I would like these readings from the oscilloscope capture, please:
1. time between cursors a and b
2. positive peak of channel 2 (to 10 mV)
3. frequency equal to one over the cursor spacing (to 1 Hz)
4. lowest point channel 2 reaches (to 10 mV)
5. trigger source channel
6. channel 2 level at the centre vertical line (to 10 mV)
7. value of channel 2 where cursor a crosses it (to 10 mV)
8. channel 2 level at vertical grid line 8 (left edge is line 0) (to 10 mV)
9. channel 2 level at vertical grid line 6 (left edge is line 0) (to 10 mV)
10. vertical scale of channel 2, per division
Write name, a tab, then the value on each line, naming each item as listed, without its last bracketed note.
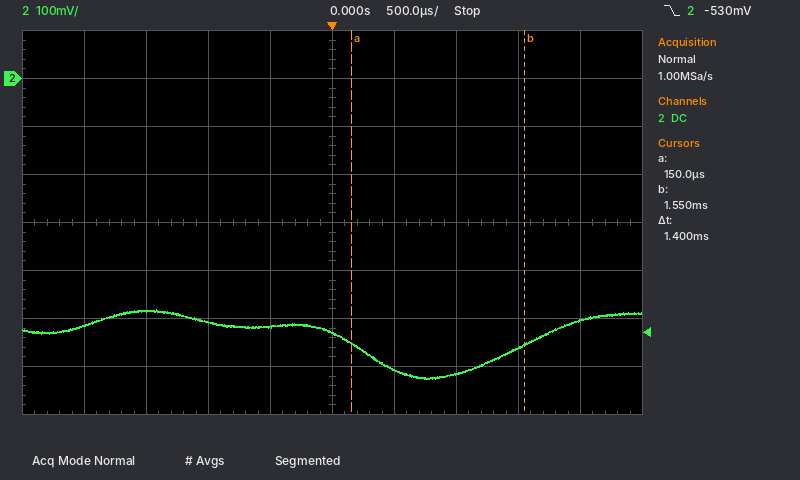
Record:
time between cursors a and b	1.4 ms
positive peak of channel 2	-480 mV
frequency equal to one over the cursor spacing	714 Hz
lowest point channel 2 reaches	-630 mV
trigger source channel	channel 2
channel 2 level at the centre vertical line	-530 mV
value of channel 2 where cursor a crosses it	-550 mV
channel 2 level at vertical grid line 8 (left edge is line 0)	-560 mV
channel 2 level at vertical grid line 6 (left edge is line 0)	-610 mV
vertical scale of channel 2, per division	100 mV
